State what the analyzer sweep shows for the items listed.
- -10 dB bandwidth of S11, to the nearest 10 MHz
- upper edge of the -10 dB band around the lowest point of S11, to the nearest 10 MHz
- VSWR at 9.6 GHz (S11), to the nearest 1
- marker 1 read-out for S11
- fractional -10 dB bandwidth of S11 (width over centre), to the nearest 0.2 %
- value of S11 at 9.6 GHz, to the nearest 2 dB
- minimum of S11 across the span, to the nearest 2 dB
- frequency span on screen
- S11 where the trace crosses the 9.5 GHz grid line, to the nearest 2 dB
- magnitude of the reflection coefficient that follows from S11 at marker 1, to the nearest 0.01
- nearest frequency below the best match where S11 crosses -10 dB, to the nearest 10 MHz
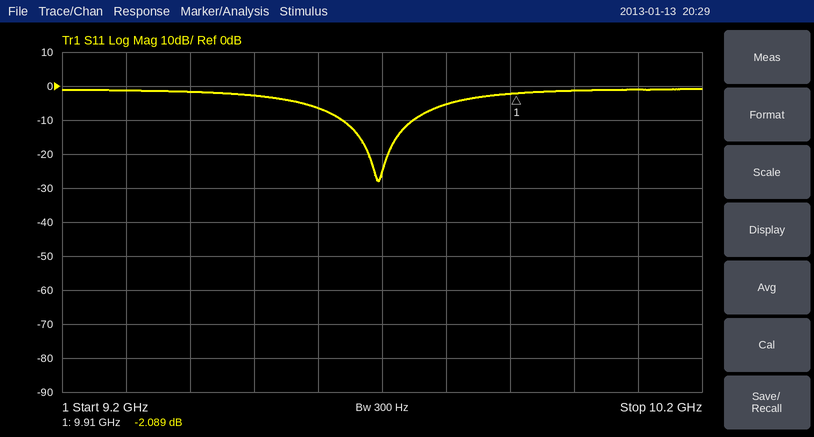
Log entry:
110 MHz
9.75 GHz
3
-2.089 dB
1.2 %
-6 dB
-28 dB
1 GHz
-2 dB
0.79
9.64 GHz
